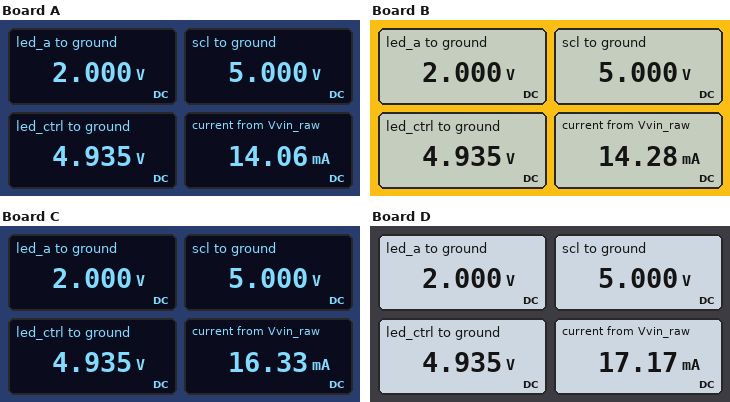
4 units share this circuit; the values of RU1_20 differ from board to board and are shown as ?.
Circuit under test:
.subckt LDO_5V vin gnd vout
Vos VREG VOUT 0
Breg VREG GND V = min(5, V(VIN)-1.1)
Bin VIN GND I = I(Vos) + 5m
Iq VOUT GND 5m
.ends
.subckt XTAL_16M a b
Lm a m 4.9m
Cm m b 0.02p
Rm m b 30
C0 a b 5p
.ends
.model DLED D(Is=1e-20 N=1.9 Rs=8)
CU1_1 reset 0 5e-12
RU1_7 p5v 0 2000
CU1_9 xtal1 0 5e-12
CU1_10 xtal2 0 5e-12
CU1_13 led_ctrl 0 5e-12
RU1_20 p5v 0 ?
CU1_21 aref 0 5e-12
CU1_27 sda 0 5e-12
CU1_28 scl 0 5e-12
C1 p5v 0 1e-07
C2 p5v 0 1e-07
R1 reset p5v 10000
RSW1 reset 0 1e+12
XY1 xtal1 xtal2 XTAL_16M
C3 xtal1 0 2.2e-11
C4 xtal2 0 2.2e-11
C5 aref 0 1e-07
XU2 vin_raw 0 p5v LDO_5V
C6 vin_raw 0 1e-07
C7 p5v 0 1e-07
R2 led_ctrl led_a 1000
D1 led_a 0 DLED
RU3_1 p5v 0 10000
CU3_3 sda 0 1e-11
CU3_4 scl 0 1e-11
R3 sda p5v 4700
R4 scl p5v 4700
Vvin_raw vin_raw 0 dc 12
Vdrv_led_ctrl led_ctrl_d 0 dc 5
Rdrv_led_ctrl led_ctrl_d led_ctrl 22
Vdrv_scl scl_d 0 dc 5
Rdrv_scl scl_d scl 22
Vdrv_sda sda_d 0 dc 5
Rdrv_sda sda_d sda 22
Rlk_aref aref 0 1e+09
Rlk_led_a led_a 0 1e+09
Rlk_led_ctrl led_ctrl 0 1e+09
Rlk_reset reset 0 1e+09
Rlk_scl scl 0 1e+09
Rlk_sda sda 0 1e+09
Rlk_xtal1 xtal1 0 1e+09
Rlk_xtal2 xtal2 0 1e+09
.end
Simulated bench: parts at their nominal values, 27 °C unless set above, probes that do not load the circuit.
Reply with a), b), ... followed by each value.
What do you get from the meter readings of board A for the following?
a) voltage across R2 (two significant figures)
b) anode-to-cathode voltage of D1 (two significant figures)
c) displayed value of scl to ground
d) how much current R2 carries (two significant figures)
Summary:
a) 2.9 V
b) 2.0 V
c) 5.000 V
d) 2.9 mA
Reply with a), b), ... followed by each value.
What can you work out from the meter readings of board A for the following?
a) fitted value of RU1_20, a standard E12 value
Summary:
a) 4.7 kΩ
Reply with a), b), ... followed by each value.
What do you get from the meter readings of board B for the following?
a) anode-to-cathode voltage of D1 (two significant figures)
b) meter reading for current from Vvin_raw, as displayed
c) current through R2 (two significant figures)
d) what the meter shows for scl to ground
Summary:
a) 2.0 V
b) 14.28 mA
c) 2.9 mA
d) 5.000 V
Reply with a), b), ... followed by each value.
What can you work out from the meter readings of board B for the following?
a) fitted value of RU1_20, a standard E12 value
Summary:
a) 3.9 kΩ
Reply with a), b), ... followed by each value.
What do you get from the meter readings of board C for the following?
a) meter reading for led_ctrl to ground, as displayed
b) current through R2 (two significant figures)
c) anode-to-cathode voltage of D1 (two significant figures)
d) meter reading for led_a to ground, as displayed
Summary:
a) 4.935 V
b) 2.9 mA
c) 2.0 V
d) 2.000 V
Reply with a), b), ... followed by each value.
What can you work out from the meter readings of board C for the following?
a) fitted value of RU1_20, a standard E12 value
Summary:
a) 1.5 kΩ
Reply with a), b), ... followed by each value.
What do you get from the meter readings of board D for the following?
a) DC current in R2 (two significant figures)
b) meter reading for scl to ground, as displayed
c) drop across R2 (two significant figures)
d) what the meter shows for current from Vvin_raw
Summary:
a) 2.9 mA
b) 5.000 V
c) 2.9 V
d) 17.17 mA
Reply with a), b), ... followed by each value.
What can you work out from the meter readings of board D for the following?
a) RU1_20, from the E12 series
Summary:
a) 1.2 kΩ
